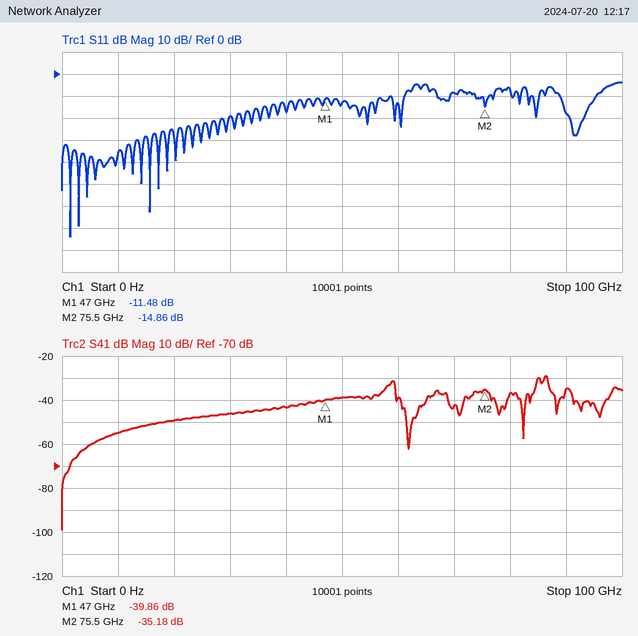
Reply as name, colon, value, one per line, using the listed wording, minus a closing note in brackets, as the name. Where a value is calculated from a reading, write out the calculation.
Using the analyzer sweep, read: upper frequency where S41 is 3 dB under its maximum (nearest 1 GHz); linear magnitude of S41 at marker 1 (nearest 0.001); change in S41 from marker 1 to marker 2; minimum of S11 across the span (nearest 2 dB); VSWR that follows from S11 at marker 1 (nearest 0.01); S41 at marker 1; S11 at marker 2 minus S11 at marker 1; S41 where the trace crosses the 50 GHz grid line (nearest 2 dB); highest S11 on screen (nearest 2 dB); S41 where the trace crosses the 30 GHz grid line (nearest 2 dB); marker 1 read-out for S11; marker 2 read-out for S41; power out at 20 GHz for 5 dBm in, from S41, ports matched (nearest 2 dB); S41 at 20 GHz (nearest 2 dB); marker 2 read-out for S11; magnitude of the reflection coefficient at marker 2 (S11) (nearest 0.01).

upper frequency where S41 is 3 dB under its maximum: 87 GHz
linear magnitude of S41 at marker 1: 10^(-39.86/20) ≈ 0.010
change in S41 from marker 1 to marker 2: -35.18 − (-39.86) = 4.68 dB
minimum of S11 across the span: -74 dB
VSWR that follows from S11 at marker 1: (1 + 0.2667)/(1 − 0.2667) ≈ 1.73
S41 at marker 1: -39.86 dB
S11 at marker 2 minus S11 at marker 1: -14.86 − (-11.48) = -3.38 dB
S41 where the trace crosses the 50 GHz grid line: -38 dB
highest S11 on screen: -4 dB
S41 where the trace crosses the 30 GHz grid line: -46 dB
marker 1 read-out for S11: -11.48 dB
marker 2 read-out for S41: -35.18 dB
power out at 20 GHz for 5 dBm in, from S41, ports matched: 5 dBm + (-50 dB) = -44 dBm
S41 at 20 GHz: -50 dB
marker 2 read-out for S11: -14.86 dB
magnitude of the reflection coefficient at marker 2 (S11): 10^(-14.86/20) ≈ 0.18
